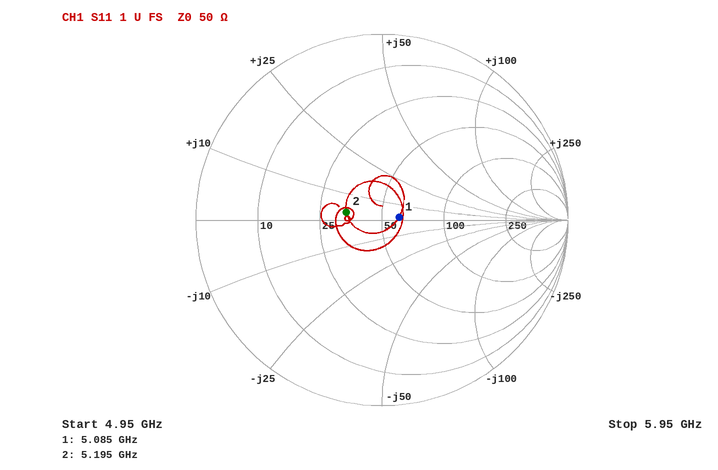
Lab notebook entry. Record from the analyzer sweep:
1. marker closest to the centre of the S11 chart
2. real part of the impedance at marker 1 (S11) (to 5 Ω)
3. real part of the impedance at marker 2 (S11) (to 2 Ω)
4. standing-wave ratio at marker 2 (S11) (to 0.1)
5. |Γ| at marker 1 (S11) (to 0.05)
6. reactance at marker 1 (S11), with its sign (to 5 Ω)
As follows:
marker 1
60 Ω
34 Ω
1.5
0.10
0 Ω
